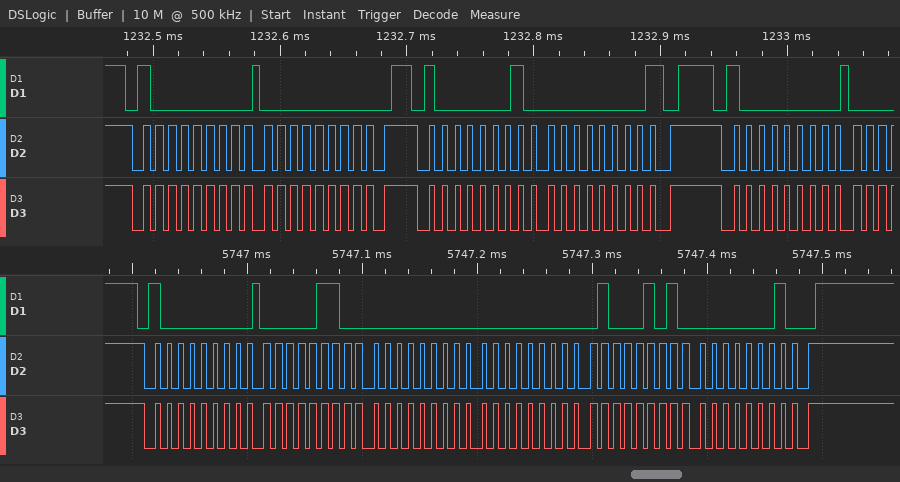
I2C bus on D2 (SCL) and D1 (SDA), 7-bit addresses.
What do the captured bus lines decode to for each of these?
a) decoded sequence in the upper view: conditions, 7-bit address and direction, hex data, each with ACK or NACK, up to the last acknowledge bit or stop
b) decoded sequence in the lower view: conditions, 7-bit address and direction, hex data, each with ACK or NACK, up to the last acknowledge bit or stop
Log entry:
start, address 40 write ACK, 00 ACK, stop, start, address 40 read ACK, 00 NACK, stop, start, address 40 write ACK
start, address 40 write ACK, 06 ACK, 00 ACK, 00 ACK, 45 ACK, 01 ACK, stop
